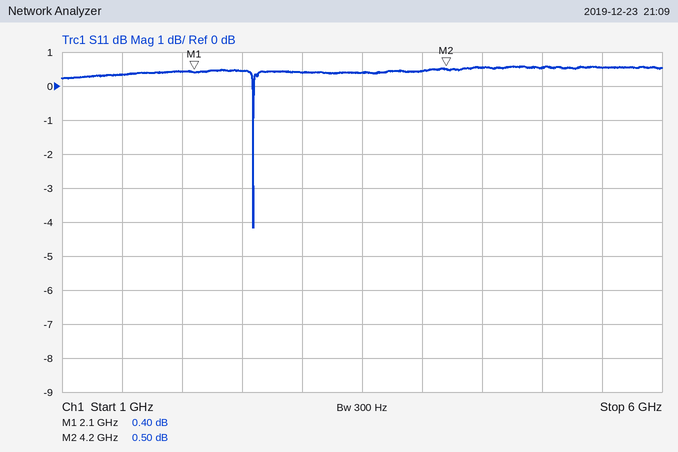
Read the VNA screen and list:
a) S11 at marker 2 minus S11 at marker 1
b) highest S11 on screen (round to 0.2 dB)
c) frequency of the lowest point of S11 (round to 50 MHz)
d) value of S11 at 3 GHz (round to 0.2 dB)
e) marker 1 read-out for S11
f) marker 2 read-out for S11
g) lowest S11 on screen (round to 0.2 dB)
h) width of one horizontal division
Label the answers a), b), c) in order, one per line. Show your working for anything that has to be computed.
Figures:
a) 0.5 − (0.4) = 0.10 dB
b) 0.6 dB
c) 2.60 GHz
d) 0.4 dB
e) 0.40 dB
f) 0.50 dB
g) -4.2 dB
h) 500 MHz
